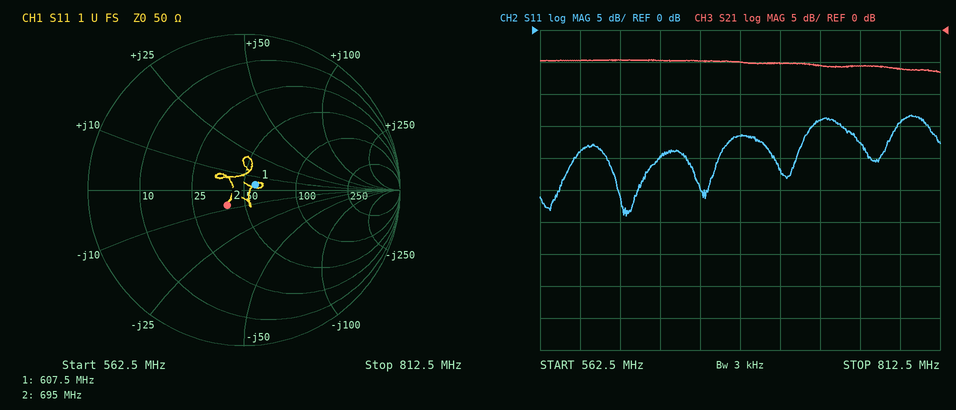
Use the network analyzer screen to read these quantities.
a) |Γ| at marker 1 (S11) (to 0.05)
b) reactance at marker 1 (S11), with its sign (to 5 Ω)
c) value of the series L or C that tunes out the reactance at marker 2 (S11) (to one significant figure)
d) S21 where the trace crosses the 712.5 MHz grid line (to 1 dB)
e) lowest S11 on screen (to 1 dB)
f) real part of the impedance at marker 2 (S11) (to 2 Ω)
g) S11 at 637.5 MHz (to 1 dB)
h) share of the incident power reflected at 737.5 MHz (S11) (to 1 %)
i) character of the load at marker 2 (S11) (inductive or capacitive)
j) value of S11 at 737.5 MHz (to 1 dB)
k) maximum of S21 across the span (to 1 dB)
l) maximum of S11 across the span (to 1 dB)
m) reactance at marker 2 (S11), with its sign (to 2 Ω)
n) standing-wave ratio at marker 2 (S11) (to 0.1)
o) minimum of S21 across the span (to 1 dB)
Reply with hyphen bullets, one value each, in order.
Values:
- 0.10
- +5 Ω
- 2 nH
- -5 dB
- -29 dB
- 40 Ω
- -20 dB
- 4 %
- capacitive
- -14 dB
- -5 dB
- -13 dB
- -8 Ω
- 1.3
- -7 dB
